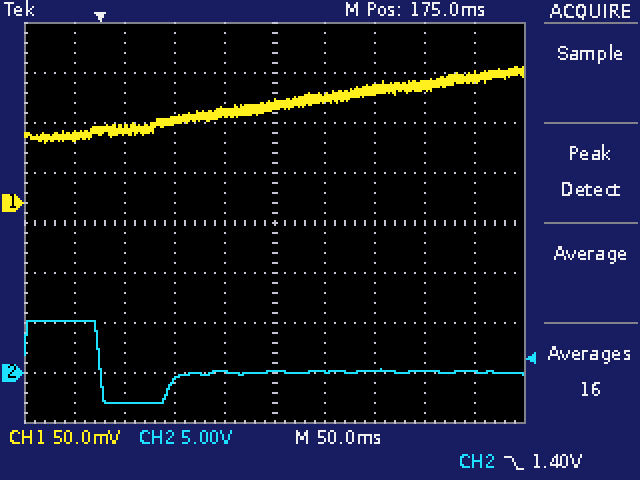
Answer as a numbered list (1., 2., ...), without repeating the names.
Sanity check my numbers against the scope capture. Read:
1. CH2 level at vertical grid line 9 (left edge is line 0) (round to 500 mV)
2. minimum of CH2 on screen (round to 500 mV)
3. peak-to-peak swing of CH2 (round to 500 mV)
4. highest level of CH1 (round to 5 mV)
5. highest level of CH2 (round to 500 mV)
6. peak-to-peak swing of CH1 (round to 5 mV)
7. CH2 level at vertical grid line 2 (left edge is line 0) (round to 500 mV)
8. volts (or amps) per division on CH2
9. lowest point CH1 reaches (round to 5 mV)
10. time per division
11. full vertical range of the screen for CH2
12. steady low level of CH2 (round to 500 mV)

1. 0.0 V
2. -3.0 V
3. 8.0 V
4. 135 mV
5. 5.0 V
6. 75 mV
7. -3.0 V
8. 5 V
9. 60 mV
10. 50 ms
11. 40 V
12. 0.0 V
